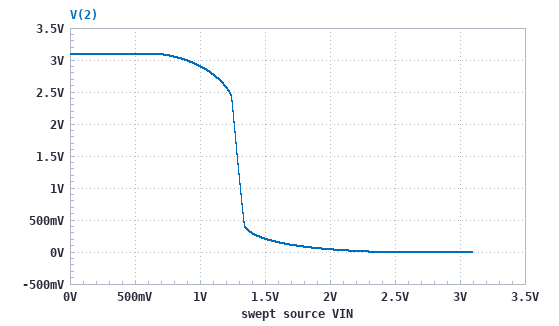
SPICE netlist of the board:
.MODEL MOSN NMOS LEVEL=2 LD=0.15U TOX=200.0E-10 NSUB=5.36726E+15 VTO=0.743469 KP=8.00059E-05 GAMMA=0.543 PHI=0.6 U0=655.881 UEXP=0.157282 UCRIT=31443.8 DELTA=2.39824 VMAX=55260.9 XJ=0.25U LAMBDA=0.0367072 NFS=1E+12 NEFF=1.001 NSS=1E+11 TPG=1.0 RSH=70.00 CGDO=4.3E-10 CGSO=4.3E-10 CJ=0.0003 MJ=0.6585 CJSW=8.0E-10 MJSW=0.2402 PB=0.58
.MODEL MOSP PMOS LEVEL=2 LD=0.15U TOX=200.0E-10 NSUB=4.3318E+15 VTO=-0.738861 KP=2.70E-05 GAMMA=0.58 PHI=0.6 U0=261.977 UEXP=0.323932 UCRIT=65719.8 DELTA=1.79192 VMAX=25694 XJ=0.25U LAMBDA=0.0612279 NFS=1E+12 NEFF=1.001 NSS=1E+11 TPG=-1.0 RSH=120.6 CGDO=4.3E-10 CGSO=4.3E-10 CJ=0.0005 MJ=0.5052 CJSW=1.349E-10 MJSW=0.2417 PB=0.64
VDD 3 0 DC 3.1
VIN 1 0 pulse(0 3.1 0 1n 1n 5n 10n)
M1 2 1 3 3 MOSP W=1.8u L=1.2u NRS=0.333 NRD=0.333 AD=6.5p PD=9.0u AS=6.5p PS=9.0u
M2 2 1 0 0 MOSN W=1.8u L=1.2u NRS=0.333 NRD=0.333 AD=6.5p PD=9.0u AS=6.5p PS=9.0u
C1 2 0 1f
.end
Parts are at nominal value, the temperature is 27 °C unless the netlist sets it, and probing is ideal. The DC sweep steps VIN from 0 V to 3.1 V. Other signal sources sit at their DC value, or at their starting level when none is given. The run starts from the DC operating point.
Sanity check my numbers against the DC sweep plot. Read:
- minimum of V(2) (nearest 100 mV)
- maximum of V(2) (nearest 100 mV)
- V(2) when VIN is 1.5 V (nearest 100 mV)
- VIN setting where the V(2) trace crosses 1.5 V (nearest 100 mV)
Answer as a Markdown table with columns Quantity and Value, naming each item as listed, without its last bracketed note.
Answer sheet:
| Quantity | Value |
|---|---|
| minimum of V(2) | 0 V |
| maximum of V(2) | 3.1 V |
| V(2) when VIN is 1.5 V | 200 mV |
| VIN setting where the V(2) trace crosses 1.5 V | 1.3 V |
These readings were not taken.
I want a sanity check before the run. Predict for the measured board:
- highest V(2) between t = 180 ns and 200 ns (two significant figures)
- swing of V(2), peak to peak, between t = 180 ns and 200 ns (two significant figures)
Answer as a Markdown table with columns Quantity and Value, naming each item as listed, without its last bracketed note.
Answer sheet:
| Quantity | Value |
|---|---|
| highest V(2) between t = 180 ns and 200 ns | 3.2 V |
| swing of V(2), peak to peak, between t = 180 ns and 200 ns | 3.2 V |
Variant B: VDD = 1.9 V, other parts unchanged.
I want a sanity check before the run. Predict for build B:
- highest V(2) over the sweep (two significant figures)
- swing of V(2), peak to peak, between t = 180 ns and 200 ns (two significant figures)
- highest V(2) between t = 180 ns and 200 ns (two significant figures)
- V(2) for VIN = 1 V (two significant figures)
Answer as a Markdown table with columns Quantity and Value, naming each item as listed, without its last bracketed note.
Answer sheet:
| Quantity | Value |
|---|---|
| highest V(2) over the sweep | 1.9 V |
| swing of V(2), peak to peak, between t = 180 ns and 200 ns | 2.1 V |
| highest V(2) between t = 180 ns and 200 ns | 2.0 V |
| V(2) for VIN = 1 V | 51 mV |
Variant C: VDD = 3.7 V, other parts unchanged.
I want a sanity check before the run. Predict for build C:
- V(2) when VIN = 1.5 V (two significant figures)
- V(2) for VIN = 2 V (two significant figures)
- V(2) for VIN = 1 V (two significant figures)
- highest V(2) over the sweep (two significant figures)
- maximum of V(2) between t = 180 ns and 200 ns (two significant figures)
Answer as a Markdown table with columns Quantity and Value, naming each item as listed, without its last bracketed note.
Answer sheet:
| Quantity | Value |
|---|---|
| V(2) when VIN = 1.5 V | 1.4 V |
| V(2) for VIN = 2 V | 160 mV |
| V(2) for VIN = 1 V | 3.5 V |
| highest V(2) over the sweep | 3.7 V |
| maximum of V(2) between t = 180 ns and 200 ns | 3.8 V |
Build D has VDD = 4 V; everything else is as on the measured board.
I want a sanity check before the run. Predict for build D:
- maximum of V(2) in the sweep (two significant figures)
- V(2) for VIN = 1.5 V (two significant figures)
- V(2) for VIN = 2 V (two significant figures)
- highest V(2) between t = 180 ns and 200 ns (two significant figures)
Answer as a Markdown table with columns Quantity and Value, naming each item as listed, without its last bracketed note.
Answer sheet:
| Quantity | Value |
|---|---|
| maximum of V(2) in the sweep | 4.0 V |
| V(2) for VIN = 1.5 V | 3.1 V |
| V(2) for VIN = 2 V | 240 mV |
| highest V(2) between t = 180 ns and 200 ns | 4.1 V |
